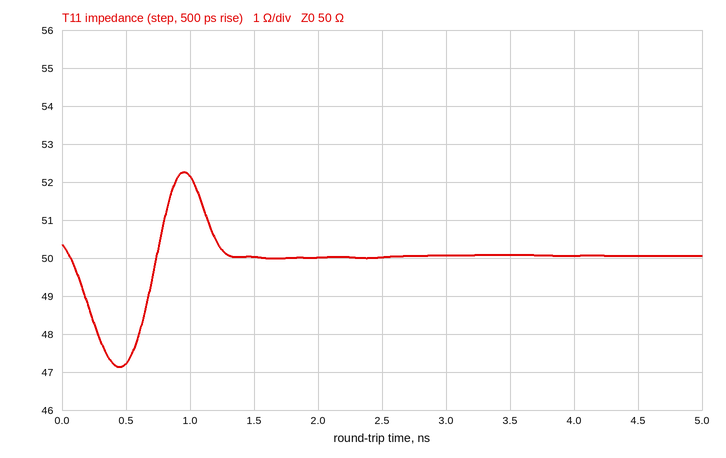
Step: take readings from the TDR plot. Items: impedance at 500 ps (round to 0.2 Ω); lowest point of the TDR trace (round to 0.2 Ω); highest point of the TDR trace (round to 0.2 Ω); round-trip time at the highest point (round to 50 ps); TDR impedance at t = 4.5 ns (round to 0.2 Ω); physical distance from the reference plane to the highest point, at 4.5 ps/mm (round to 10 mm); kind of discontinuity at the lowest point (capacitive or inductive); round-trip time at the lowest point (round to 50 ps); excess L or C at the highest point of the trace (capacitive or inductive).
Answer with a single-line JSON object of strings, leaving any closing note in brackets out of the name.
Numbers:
{"impedance at 500 ps": "47.2 Ω", "lowest point of the TDR trace": "47.2 Ω", "highest point of the TDR trace": "52.2 Ω", "round-trip time at the highest point": "950 ps", "TDR impedance at t = 4.5 ns": "50.0 Ω", "physical distance from the reference plane to the highest point, at 4.5 ps/mm": "110 mm", "kind of discontinuity at the lowest point": "capacitive", "round-trip time at the lowest point": "450 ps", "excess L or C at the highest point of the trace": "inductive"}
